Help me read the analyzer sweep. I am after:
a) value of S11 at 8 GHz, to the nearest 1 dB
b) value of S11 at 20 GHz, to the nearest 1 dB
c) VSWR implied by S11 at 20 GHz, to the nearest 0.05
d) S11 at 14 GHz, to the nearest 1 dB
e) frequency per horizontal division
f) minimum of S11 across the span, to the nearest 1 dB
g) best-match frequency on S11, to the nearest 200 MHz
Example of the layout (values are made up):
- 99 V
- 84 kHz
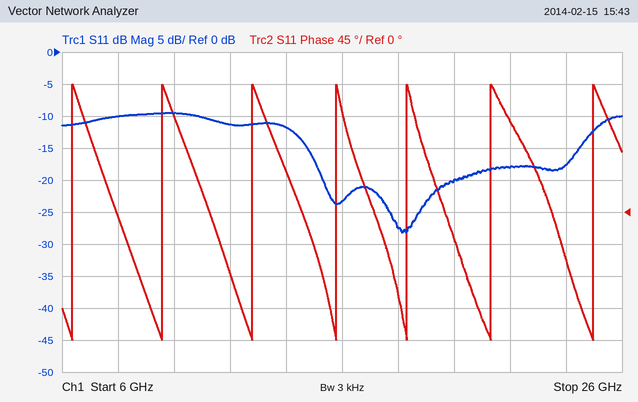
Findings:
- -10 dB
- -20 dB
- 1.20
- -12 dB
- 2 GHz
- -28 dB
- 18.2 GHz
